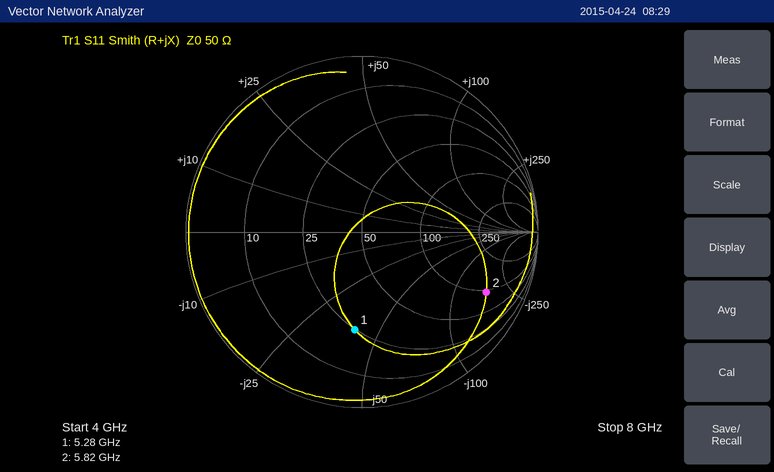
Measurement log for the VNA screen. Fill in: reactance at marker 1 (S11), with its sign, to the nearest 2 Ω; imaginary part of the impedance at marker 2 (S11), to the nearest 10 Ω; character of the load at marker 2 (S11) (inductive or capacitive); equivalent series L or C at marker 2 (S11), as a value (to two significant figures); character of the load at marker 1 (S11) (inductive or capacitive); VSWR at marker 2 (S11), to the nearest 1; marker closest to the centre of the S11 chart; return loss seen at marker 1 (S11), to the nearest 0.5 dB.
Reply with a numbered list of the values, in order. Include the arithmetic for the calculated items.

1. -40 Ω
2. -170 Ω
3. capacitive
4. C = 1/(2π × 5.82 GHz × 170 Ω) ≈ 161 fF, so 160 fF to two significant figures
5. capacitive
6. 8
7. marker 1
8. 5.0 dB
